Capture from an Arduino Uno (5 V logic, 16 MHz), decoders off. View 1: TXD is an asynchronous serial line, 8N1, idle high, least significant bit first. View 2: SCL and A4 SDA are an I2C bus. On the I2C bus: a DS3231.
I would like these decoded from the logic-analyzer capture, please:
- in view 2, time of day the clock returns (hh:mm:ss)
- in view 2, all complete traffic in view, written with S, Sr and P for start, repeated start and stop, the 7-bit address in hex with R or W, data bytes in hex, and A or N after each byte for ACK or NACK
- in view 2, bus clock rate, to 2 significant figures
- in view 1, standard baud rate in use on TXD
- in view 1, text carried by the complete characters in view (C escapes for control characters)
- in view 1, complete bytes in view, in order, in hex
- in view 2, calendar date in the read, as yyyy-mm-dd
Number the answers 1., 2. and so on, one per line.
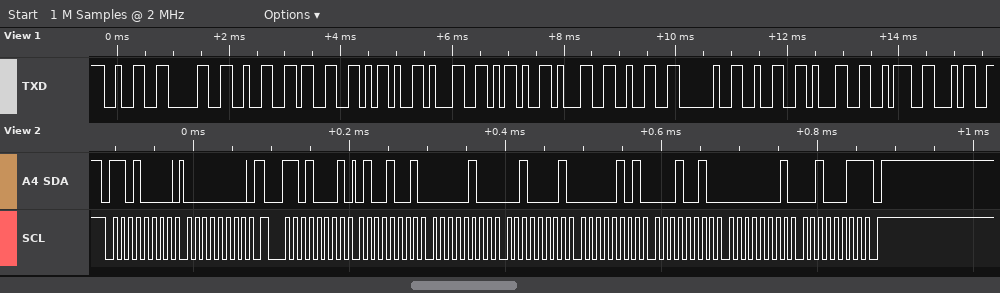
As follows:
1. 21:04:49
2. S 68W A 00 A Sr 68R A 49 A 04 A 21 A 05 A 12 A 01 A 23 N P
3. 100 kHz
4. 9600 baud
5. "2023-1-12 21:4"
6. 0x32 0x30 0x32 0x33 0x2D 0x31 0x2D 0x31 0x32 0x20 0x32 0x31 0x3A 0x34
7. 2023-01-12
